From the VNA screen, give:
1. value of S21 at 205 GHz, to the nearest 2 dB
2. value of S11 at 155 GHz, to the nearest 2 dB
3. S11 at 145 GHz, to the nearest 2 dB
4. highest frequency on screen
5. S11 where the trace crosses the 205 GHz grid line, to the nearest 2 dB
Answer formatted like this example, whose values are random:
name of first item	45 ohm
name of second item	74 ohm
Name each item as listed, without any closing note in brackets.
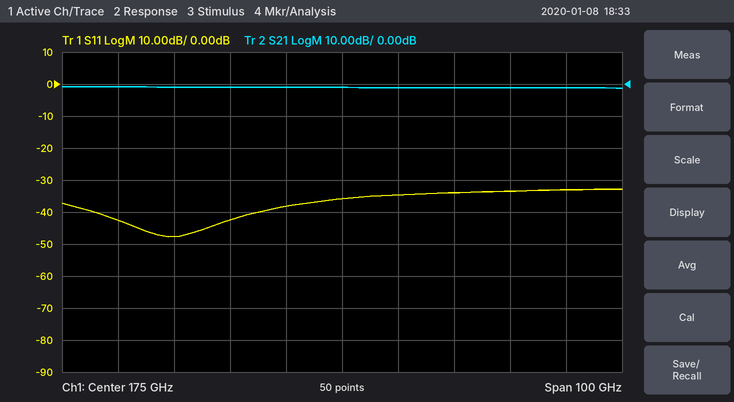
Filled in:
value of S21 at 205 GHz, to the nearest 2 dB	-2 dB
value of S11 at 155 GHz, to the nearest 2 dB	-42 dB
S11 at 145 GHz, to the nearest 2 dB	-48 dB
highest frequency on screen	225 GHz
S11 where the trace crosses the 205 GHz grid line, to the nearest 2 dB	-34 dB
